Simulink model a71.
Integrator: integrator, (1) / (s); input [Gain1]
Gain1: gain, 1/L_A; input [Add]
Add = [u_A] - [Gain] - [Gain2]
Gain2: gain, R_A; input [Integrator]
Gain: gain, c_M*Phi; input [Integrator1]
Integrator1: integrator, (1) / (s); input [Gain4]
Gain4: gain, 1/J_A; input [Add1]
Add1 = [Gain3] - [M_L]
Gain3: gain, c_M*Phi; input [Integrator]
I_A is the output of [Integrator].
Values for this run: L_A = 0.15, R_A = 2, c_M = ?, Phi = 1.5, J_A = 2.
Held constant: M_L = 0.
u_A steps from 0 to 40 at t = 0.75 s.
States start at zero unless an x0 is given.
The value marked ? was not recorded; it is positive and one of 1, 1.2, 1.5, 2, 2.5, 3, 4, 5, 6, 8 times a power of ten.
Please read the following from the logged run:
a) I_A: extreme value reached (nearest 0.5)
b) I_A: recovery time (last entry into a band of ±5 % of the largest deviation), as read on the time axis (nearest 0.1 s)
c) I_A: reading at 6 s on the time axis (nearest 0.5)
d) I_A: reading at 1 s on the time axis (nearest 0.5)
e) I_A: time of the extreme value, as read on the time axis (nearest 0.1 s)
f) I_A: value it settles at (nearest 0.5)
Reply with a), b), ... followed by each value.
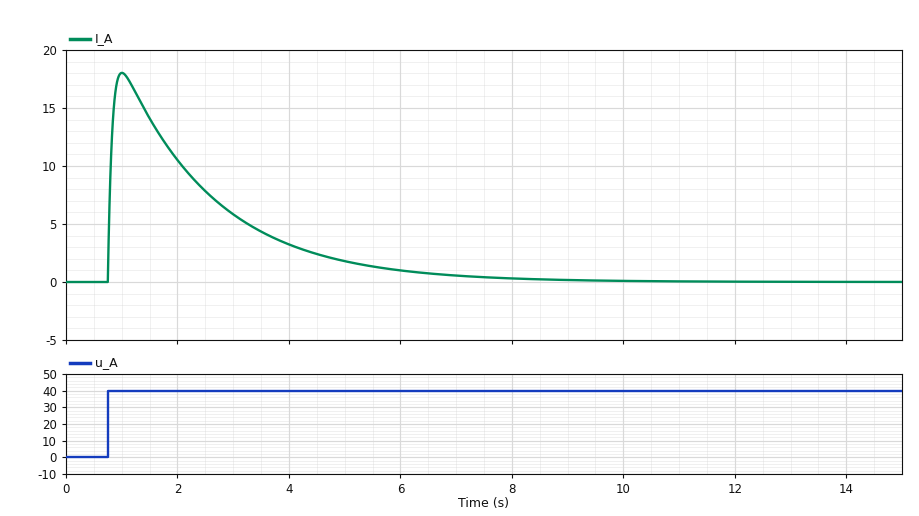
a) 18.0
b) 6.2 s
c) 1.0
d) 18.0
e) 1.0 s
f) 0.0
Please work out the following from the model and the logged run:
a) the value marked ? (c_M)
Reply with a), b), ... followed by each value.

a) 1
